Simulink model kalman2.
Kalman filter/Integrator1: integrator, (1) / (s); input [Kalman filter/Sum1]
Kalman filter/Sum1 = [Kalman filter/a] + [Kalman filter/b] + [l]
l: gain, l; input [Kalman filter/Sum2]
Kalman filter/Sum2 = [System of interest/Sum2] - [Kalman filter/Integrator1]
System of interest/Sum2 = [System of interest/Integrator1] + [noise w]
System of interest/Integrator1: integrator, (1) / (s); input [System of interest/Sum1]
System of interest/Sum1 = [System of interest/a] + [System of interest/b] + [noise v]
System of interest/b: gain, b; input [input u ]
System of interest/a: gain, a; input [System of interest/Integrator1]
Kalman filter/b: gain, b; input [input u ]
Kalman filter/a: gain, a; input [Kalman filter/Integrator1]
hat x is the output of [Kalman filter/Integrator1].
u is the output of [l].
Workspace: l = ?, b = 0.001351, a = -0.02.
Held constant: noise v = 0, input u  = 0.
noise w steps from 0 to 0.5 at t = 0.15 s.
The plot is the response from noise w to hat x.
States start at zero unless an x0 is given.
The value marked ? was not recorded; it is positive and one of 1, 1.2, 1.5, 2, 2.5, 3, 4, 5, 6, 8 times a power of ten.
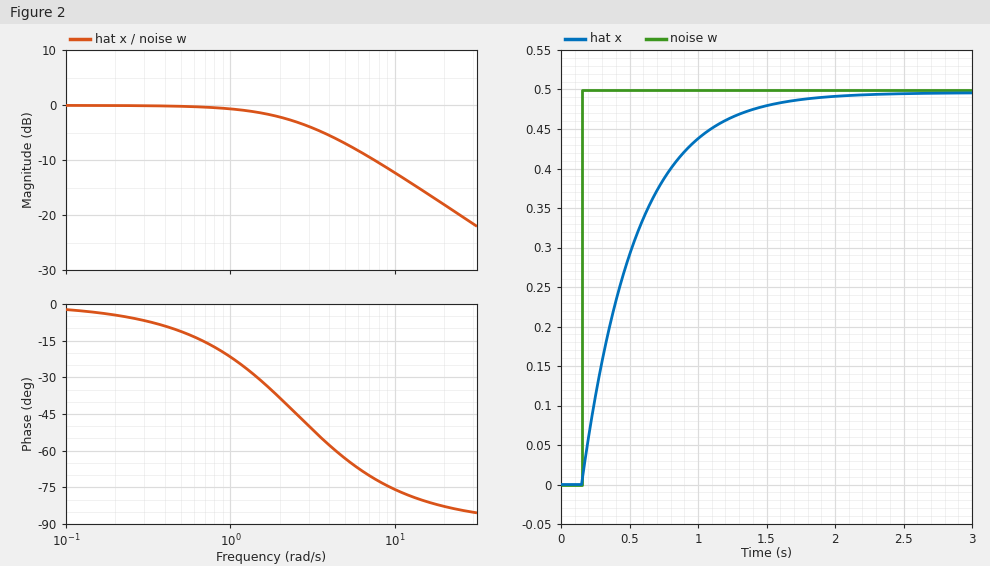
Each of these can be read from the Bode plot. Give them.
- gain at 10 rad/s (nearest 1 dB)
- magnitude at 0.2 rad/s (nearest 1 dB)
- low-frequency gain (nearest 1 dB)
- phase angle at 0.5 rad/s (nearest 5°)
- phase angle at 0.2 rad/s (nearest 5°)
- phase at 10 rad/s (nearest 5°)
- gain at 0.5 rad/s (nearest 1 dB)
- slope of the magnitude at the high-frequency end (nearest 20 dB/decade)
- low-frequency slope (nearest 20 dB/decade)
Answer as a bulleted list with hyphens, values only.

- -12 dB
- 0 dB
- 0 dB
- -10°
- -5°
- -75°
- 0 dB
- -20 dB/decade
- 0 dB/decade
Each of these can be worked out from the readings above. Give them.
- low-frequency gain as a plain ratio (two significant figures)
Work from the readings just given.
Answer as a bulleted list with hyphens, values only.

- 1.0
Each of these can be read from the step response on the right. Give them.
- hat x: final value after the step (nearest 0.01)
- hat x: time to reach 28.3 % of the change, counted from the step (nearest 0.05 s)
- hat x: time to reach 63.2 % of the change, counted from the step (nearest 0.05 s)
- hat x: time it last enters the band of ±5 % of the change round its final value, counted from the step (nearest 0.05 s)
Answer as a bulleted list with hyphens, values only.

- 0.50
- 0.15 s
- 0.40 s
- 1.20 s
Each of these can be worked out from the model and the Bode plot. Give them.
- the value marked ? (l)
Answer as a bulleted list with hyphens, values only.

- 2.5
